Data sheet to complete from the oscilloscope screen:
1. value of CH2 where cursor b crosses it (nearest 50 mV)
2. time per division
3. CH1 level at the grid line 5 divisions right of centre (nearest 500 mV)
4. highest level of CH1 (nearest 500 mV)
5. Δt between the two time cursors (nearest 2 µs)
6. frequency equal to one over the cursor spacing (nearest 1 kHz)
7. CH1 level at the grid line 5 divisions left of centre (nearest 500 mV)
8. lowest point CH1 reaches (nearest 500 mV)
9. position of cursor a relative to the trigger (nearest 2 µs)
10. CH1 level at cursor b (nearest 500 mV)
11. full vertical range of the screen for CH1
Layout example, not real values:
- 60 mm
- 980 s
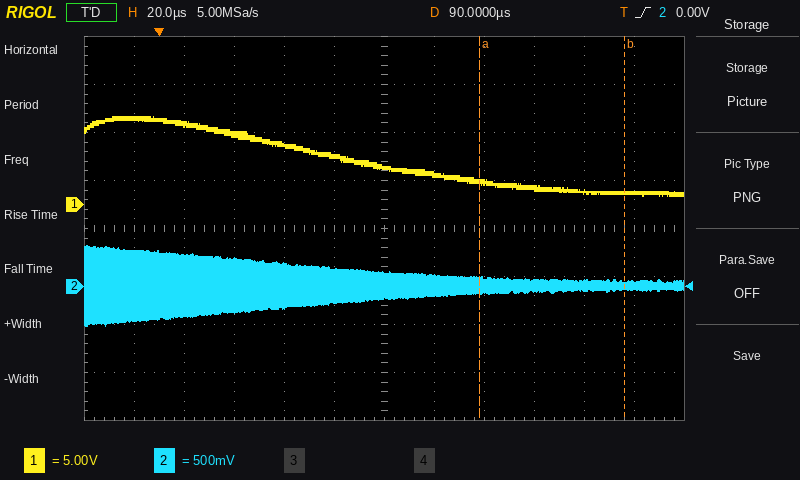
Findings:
- 0 mV
- 20 µs
- 1.0 V
- 9.0 V
- 58 µs
- 17 kHz
- 9.0 V
- 1.0 V
- +128 µs
- 1.0 V
- 40 V
